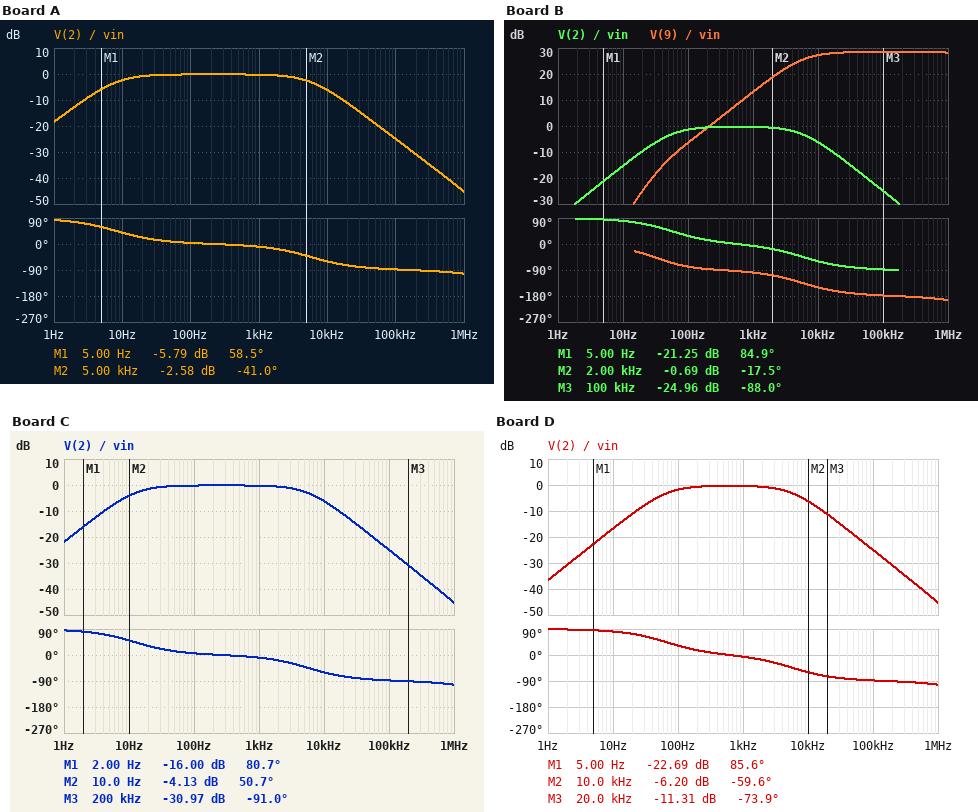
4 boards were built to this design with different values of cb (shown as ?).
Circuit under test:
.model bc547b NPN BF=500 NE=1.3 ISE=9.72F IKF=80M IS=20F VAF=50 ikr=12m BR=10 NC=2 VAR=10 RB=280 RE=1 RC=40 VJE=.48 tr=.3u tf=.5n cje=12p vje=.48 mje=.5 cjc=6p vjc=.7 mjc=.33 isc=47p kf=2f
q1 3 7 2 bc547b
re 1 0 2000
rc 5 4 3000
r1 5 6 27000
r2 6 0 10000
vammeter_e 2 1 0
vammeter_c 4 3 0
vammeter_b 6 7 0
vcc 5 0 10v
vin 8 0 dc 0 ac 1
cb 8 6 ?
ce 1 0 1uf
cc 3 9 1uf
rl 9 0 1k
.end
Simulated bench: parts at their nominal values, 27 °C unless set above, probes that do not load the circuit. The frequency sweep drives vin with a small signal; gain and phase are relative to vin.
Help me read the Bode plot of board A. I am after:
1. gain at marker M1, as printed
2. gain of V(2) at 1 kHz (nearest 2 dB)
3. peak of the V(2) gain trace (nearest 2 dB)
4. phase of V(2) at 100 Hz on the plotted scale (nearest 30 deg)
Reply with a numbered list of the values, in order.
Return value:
1. -5.79 dB
2. 0 dB
3. 0 dB
4. 0 deg
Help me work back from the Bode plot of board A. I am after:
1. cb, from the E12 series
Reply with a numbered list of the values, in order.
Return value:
1. 2.7 µF
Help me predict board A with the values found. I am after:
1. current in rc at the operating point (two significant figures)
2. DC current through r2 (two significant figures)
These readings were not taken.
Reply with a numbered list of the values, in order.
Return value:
1. 1.0 mA
2. 270 µA
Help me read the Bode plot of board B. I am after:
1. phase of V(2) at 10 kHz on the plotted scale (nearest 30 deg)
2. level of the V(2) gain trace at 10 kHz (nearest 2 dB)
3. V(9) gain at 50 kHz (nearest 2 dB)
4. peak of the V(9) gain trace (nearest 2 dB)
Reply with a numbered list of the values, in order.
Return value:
1. -60 deg
2. -6 dB
3. 28 dB
4. 28 dB
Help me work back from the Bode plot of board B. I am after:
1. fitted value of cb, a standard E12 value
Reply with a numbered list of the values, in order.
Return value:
1. 390 nF
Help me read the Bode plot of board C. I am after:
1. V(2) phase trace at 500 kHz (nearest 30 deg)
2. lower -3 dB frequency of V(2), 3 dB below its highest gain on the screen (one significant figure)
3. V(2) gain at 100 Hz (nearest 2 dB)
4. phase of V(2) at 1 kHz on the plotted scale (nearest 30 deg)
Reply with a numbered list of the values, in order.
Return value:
1. -90 deg
2. 10 Hz
3. 0 dB
4. 0 deg
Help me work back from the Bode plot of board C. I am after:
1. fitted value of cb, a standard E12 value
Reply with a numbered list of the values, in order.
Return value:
1. 1.8 µF
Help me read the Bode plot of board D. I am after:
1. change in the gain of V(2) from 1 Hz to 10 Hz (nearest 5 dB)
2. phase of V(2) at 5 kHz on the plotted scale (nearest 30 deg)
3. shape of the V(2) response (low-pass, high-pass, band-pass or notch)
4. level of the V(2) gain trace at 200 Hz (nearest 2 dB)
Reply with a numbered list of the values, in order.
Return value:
1. 20 dB
2. -30 deg
3. band-pass
4. 0 dB
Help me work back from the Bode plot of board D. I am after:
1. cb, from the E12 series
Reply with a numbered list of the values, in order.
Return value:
1. 330 nF
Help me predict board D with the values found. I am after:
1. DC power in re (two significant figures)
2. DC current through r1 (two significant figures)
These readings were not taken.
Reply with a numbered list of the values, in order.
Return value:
1. 2.1 mW
2. 270 µA
